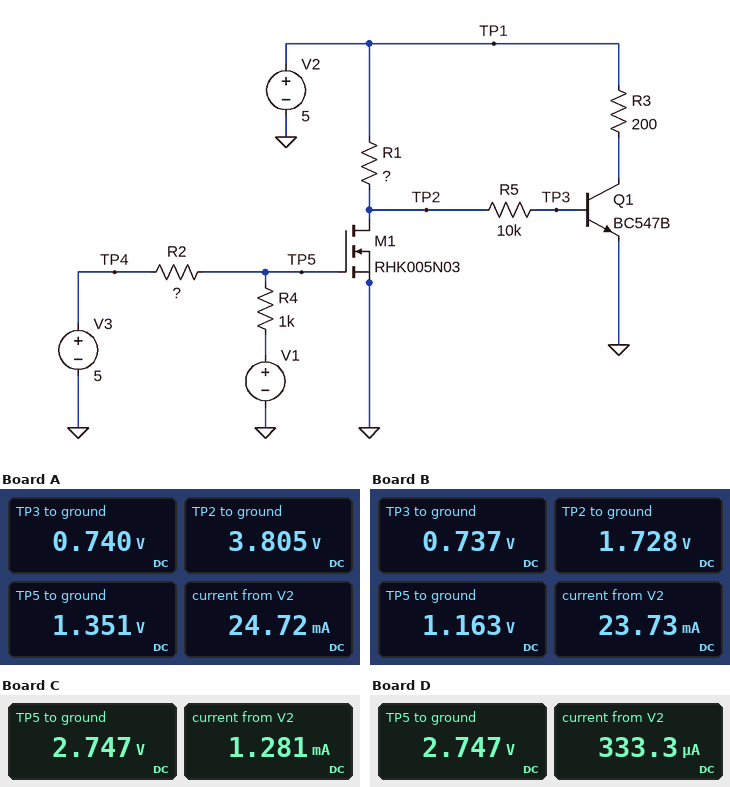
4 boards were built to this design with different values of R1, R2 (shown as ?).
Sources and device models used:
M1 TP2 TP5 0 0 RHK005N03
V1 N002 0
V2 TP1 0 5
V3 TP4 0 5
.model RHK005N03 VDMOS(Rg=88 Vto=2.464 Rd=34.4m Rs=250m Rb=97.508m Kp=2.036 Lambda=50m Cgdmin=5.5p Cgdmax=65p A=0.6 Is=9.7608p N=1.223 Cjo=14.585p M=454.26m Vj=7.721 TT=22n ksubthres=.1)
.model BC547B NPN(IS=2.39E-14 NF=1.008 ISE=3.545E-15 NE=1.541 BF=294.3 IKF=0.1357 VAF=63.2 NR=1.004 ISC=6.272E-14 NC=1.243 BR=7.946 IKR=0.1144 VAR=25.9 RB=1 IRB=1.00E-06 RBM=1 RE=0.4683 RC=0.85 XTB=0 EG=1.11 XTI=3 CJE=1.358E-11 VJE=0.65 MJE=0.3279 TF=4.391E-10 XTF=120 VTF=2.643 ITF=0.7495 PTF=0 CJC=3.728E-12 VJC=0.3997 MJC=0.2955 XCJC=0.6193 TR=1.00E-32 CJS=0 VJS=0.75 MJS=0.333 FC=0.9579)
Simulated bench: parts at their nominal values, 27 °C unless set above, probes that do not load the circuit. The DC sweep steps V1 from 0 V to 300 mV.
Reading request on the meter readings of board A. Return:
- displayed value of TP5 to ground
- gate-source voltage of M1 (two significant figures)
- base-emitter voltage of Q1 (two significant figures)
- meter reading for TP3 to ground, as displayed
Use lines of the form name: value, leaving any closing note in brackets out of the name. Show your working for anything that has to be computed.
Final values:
displayed value of TP5 to ground: 1.351 V
gate-source voltage of M1: 1.351 V = 1.4 V
base-emitter voltage of Q1: 740 mV = 740 mV
meter reading for TP3 to ground, as displayed: 0.740 V
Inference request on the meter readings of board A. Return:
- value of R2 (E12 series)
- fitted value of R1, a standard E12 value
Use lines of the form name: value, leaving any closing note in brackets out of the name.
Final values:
value of R2: 2.7 kΩ
fitted value of R1, a standard E12 value: 3.9 kΩ
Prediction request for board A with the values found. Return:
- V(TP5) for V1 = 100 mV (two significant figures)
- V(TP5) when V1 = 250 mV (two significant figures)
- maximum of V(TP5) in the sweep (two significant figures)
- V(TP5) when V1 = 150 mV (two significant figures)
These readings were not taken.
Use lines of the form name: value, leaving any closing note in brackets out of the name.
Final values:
V(TP5) for V1 = 100 mV: 1.4 V
V(TP5) when V1 = 250 mV: 1.5 V
maximum of V(TP5) in the sweep: 1.6 V
V(TP5) when V1 = 150 mV: 1.5 V
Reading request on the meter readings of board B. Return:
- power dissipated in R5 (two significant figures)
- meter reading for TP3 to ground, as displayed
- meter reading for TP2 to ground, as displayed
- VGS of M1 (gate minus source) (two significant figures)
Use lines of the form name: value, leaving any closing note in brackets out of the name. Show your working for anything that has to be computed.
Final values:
power dissipated in R5: (1.728 V - 737 mV)^2 / 10 kΩ = 98 µW
meter reading for TP3 to ground, as displayed: 0.737 V
meter reading for TP2 to ground, as displayed: 1.728 V
VGS of M1 (gate minus source): 1.163 V = 1.2 V
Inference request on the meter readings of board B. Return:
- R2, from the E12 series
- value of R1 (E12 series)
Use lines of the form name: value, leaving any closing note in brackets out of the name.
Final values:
R2, from the E12 series: 3.3 kΩ
value of R1: 33 kΩ
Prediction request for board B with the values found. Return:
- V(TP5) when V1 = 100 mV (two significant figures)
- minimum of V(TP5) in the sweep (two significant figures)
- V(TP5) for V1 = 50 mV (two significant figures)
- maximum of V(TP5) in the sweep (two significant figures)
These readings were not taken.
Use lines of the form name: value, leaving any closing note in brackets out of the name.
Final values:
V(TP5) when V1 = 100 mV: 1.2 V
minimum of V(TP5) in the sweep: 1.2 V
V(TP5) for V1 = 50 mV: 1.2 V
maximum of V(TP5) in the sweep: 1.4 V
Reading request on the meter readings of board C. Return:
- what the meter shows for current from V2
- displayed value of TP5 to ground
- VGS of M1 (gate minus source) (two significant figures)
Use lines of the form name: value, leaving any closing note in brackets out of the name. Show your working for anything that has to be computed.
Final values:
what the meter shows for current from V2: 1.281 mA
displayed value of TP5 to ground: 2.747 V
VGS of M1 (gate minus source): 2.747 V = 2.7 V
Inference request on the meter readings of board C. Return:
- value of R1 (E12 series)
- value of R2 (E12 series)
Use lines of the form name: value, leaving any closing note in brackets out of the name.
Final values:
value of R1: 3.9 kΩ
value of R2: 820 Ω
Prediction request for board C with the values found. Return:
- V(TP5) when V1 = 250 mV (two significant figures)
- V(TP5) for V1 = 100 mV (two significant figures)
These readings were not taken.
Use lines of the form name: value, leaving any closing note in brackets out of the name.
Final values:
V(TP5) when V1 = 250 mV: 2.9 V
V(TP5) for V1 = 100 mV: 2.8 V
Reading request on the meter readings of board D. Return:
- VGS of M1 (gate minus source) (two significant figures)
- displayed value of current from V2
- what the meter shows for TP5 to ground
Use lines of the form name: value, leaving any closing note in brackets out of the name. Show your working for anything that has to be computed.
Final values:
VGS of M1 (gate minus source): 2.747 V = 2.7 V
displayed value of current from V2: 333.3 µA
what the meter shows for TP5 to ground: 2.747 V
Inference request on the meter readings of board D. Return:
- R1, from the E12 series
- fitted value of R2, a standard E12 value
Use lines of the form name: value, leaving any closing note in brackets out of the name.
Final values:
R1, from the E12 series: 15 kΩ
fitted value of R2, a standard E12 value: 820 Ω
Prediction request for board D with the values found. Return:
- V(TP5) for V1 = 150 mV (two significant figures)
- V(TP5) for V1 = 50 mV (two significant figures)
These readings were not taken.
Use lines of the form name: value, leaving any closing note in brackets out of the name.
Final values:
V(TP5) for V1 = 150 mV: 2.8 V
V(TP5) for V1 = 50 mV: 2.8 V
